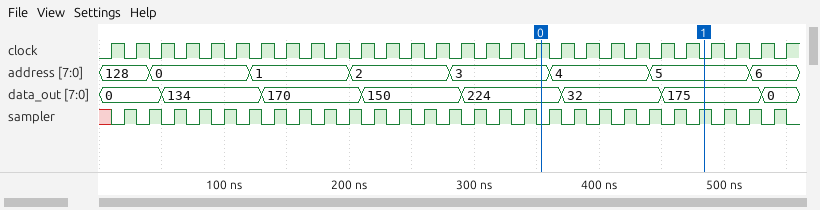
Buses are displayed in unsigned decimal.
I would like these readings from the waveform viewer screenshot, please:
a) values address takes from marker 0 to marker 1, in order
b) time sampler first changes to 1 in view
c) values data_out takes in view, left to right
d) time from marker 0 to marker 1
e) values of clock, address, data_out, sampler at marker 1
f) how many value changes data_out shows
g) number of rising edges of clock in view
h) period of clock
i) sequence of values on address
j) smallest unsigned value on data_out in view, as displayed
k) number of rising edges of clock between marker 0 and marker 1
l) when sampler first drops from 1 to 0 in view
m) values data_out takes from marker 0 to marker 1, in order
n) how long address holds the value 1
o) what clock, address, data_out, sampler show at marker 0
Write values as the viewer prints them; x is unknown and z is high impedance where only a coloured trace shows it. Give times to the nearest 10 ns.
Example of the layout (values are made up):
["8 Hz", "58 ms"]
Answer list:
["3, 4, 5", "20 ns", "0, 134, 170, 150, 224, 32, 175, 0", "130 ns", "clock=0, address=5, data_out=175, sampler=1", "7", "28", "20 ns", "128, 0, 1, 2, 3, 4, 5, 6", "0", "6", "30 ns", "224, 32, 175", "80 ns", "clock=1, address=3, data_out=224, sampler=0"]
